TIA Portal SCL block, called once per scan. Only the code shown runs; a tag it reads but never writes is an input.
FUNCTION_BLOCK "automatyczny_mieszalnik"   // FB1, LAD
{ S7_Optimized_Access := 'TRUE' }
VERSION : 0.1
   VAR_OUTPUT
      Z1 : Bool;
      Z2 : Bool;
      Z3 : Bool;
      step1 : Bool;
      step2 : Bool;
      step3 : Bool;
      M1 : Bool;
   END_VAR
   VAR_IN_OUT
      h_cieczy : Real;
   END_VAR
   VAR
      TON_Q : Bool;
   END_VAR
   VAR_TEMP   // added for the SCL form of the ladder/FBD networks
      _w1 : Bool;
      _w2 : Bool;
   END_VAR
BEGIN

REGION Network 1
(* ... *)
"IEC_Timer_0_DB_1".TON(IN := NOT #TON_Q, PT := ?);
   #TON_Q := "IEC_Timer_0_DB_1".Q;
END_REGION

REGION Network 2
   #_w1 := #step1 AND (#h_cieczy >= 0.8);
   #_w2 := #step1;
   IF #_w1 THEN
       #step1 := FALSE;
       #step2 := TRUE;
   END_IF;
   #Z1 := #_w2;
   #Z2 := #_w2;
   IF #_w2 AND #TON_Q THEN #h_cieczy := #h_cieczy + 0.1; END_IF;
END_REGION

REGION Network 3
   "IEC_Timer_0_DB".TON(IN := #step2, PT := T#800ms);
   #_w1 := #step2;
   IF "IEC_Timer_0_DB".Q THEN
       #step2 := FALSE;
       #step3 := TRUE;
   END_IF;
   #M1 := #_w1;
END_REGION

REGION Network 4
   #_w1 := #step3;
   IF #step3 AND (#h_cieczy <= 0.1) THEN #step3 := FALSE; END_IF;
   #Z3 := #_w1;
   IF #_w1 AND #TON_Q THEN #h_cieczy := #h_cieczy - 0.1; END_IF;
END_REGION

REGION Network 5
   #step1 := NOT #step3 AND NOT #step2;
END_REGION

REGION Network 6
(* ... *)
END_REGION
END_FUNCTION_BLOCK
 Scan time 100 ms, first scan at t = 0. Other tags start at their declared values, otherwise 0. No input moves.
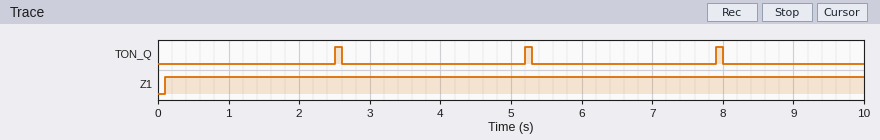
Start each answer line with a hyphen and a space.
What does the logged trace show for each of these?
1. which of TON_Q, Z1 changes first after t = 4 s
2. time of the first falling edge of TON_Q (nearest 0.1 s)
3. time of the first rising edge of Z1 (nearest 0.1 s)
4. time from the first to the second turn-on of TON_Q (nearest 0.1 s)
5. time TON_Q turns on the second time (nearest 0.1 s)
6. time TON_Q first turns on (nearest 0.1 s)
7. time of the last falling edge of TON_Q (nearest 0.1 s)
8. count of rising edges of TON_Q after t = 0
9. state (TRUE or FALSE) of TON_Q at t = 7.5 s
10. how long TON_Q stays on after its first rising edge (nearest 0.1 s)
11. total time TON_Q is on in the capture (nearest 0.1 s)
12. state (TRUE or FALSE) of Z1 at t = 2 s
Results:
- TON_Q
- 2.6 s
- 0.1 s
- 2.7 s
- 5.2 s
- 2.5 s
- 8.0 s
- 3
- FALSE
- 0.1 s
- 0.3 s
- TRUE
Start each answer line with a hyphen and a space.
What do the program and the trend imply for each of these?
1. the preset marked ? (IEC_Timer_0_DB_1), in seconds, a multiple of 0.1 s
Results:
- 2.5 s
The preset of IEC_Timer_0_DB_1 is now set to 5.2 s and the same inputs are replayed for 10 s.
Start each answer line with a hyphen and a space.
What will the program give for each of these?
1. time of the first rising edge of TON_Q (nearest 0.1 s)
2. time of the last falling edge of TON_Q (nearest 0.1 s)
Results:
- 5.2 s
- 5.3 s
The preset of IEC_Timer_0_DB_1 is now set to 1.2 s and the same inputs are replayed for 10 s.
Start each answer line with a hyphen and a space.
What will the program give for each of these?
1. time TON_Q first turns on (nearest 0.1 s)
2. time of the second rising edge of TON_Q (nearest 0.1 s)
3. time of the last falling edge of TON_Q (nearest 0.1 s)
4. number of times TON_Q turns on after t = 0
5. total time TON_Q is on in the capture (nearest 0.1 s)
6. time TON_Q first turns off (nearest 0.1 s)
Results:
- 1.2 s
- 2.6 s
- 9.7 s
- 7
- 0.7 s
- 1.3 s
